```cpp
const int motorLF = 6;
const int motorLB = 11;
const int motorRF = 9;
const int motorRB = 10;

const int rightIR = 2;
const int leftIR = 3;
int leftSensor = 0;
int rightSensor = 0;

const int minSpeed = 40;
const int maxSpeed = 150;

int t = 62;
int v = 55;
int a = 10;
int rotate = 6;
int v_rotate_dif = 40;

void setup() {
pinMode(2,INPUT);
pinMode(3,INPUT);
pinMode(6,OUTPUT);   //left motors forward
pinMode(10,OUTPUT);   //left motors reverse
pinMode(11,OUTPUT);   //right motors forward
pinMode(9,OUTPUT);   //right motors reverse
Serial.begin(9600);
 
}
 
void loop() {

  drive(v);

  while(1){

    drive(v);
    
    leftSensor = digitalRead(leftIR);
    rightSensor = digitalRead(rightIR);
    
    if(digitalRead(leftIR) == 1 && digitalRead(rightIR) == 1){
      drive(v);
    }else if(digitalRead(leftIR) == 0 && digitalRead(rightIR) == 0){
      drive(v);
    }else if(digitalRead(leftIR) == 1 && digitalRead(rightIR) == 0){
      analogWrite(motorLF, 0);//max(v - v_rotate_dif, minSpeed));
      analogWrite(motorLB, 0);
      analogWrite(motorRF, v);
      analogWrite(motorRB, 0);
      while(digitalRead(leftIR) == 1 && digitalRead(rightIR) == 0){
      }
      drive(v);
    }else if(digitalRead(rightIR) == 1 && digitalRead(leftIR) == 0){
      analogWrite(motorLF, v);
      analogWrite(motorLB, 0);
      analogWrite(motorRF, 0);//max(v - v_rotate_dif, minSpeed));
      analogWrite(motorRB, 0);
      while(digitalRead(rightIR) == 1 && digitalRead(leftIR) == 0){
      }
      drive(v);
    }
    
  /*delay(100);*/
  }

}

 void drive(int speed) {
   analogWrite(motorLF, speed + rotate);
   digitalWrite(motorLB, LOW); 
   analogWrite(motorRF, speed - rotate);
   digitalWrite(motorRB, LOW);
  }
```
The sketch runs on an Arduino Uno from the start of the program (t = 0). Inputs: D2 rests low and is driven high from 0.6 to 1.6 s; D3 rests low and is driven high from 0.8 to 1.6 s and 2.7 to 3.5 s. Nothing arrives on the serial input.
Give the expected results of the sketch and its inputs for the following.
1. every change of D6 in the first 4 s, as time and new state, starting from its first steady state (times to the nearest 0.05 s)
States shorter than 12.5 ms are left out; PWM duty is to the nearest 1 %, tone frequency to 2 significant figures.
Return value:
0 s PWM 24 %; 0.6 s PWM 22 %; 0.8 s PWM 24 %; 2.7 s low; 3.5 s PWM 24 %
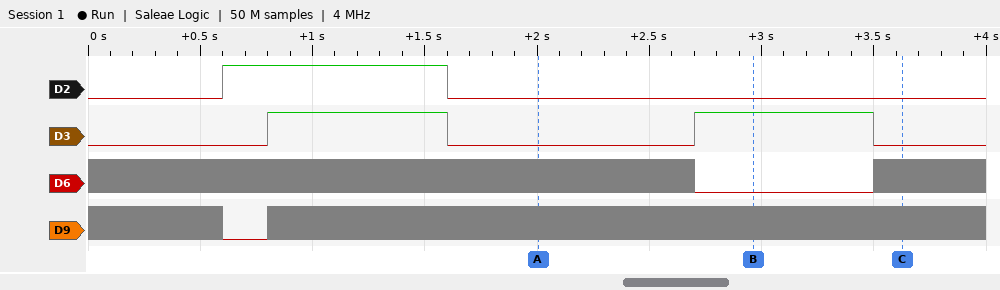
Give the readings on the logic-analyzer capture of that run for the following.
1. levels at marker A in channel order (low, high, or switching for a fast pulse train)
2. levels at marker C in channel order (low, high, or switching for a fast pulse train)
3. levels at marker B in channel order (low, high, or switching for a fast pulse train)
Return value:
D2 low, D3 low, D6 switching, D9 switching
D2 low, D3 low, D6 switching, D9 switching
D2 low, D3 high, D6 low, D9 switching
